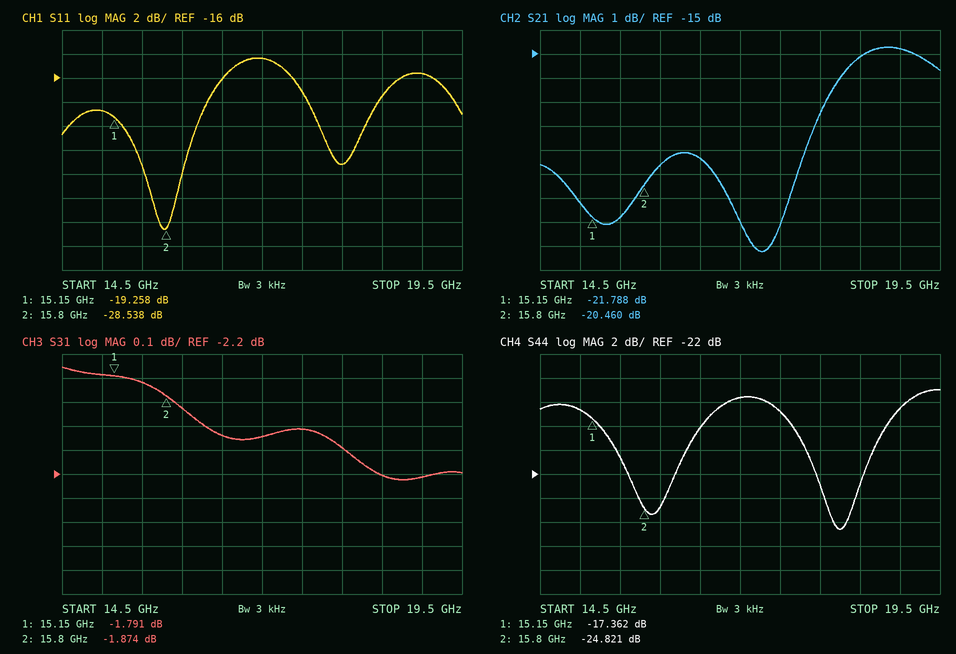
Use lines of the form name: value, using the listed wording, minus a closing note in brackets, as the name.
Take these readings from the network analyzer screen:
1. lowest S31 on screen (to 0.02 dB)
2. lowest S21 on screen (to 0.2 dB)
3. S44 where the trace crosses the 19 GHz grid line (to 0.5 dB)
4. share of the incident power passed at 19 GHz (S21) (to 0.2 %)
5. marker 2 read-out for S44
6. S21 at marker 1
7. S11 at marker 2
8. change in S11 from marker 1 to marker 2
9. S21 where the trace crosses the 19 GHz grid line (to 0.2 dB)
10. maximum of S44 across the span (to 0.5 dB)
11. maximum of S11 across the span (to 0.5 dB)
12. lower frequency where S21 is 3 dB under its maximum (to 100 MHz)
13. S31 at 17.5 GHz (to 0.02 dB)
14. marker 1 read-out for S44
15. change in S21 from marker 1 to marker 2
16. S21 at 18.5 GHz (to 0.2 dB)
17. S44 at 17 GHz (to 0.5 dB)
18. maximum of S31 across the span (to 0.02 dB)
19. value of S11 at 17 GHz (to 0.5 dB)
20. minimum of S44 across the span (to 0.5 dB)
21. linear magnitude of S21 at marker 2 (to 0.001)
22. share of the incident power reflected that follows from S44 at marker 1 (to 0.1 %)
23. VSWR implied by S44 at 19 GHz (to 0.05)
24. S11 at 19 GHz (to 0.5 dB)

lowest S31 on screen: -2.22 dB
lowest S21 on screen: -23.2 dB
S44 where the trace crosses the 19 GHz grid line: -16.5 dB
share of the incident power passed at 19 GHz (S21): 3.4 %
marker 2 read-out for S44: -24.821 dB
S21 at marker 1: -21.788 dB
S11 at marker 2: -28.538 dB
change in S11 from marker 1 to marker 2: -9.280 dB
S21 where the trace crosses the 19 GHz grid line: -14.8 dB
maximum of S44 across the span: -15.0 dB
maximum of S11 across the span: -14.5 dB
lower frequency where S21 is 3 dB under its maximum: 18.0 GHz
S31 at 17.5 GHz: -2.02 dB
marker 1 read-out for S44: -17.362 dB
change in S21 from marker 1 to marker 2: 1.328 dB
S21 at 18.5 GHz: -15.2 dB
S44 at 17 GHz: -15.5 dB
maximum of S31 across the span: -1.76 dB
value of S11 at 17 GHz: -14.5 dB
minimum of S44 across the span: -26.5 dB
linear magnitude of S21 at marker 2: 0.095
share of the incident power reflected that follows from S44 at marker 1: 1.8 %
VSWR implied by S44 at 19 GHz: 1.35
S11 at 19 GHz: -15.5 dB
